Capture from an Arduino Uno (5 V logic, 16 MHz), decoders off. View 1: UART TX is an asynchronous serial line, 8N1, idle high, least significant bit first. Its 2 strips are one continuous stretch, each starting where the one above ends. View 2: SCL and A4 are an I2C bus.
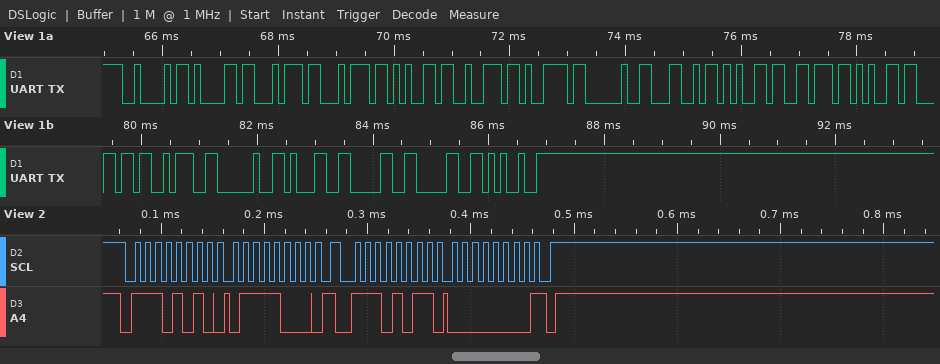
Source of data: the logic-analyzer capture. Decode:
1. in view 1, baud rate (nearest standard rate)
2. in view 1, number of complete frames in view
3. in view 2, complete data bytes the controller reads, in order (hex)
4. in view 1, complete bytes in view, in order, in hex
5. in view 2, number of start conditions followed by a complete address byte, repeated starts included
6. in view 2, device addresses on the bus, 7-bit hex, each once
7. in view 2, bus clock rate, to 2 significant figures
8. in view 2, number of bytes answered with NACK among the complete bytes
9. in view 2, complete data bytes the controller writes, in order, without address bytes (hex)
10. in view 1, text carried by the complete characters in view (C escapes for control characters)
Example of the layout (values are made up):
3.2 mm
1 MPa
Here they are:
9600 baud
19
00
0x42 0x61 0x74 0x74 0x65 0x72 0x79 0x20 0x4C 0x65 0x76 0x65 0x6C 0x3A 0x20 0x31 0x30 0x30 0x25
2
0x75
100 kHz
1
78
"Battery Level: 100%"
